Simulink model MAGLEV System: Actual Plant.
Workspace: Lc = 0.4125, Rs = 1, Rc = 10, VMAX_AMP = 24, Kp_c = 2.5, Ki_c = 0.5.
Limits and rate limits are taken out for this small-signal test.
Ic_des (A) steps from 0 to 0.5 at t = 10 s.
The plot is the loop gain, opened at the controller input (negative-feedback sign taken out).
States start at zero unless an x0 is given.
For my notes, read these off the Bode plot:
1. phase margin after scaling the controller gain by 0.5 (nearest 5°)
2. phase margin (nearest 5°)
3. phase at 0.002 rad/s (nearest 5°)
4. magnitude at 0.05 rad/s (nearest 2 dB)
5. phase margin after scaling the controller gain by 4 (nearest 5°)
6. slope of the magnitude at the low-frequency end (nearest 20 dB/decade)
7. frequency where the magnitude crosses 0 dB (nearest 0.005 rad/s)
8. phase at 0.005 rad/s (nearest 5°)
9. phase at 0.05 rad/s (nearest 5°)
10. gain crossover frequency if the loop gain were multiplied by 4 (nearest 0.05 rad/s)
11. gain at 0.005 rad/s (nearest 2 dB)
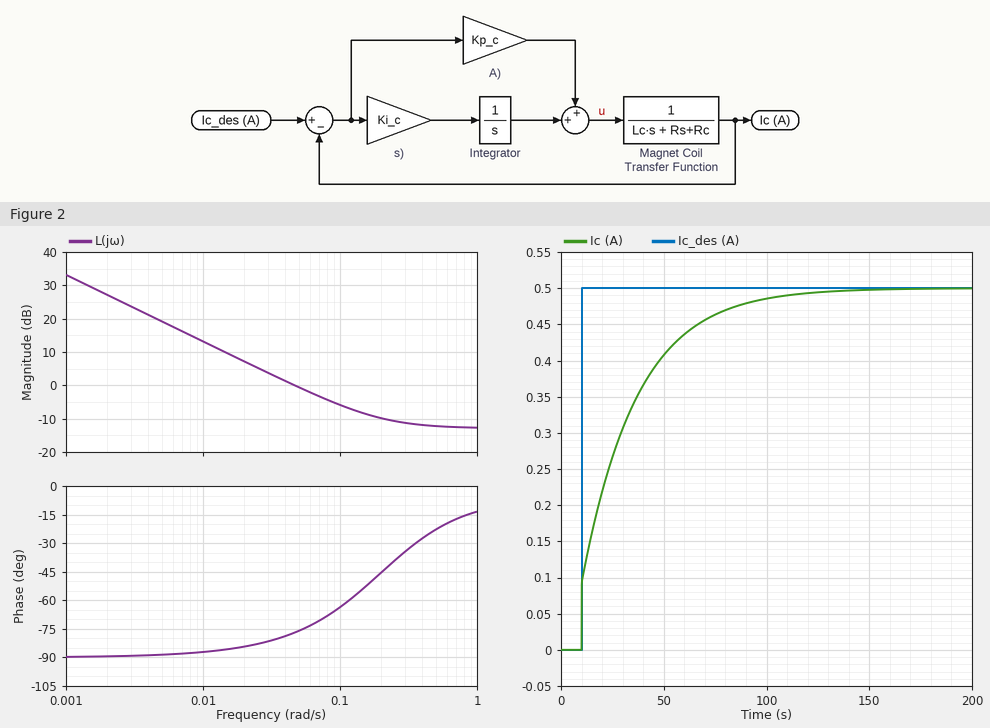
95°
105°
-90°
0 dB
155°
-20 dB/decade
0.045 rad/s
-90°
-75°
0.45 rad/s
20 dB
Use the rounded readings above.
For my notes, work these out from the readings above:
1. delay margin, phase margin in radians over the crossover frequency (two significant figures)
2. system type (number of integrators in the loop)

41 s
1
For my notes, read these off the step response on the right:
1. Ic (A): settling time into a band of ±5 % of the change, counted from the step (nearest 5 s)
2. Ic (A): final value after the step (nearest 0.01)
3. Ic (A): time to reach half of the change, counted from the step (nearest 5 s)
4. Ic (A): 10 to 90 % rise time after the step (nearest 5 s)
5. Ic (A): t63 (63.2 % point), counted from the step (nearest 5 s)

75 s
0.50
15 s
55 s
20 s
